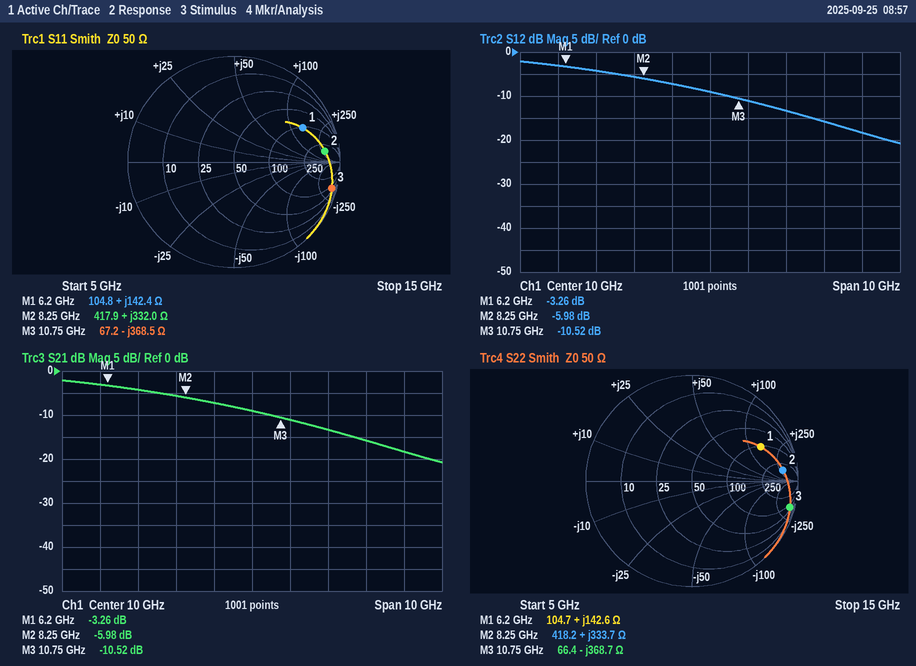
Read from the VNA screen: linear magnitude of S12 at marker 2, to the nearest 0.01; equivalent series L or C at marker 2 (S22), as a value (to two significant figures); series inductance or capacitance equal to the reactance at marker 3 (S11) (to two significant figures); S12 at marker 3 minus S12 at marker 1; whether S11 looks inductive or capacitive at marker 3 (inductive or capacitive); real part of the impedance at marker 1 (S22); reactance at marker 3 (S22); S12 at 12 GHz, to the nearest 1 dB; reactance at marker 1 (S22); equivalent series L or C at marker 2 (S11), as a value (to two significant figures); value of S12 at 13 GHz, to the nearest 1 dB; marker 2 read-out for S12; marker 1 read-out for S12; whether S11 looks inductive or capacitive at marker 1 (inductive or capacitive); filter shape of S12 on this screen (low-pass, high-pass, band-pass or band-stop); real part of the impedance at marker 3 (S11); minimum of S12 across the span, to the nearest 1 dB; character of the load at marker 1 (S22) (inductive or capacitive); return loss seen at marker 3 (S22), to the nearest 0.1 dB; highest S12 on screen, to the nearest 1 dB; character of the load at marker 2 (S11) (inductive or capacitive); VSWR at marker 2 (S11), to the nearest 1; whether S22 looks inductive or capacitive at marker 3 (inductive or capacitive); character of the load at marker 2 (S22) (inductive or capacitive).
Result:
0.50
6.4 nH
40 fF
-7.26 dB
capacitive
104.7 Ω
-368.7 Ω
-13 dB
+142.6 Ω
6.4 nH
-16 dB
-5.98 dB
-3.26 dB
inductive
low-pass
67.2 Ω
-21 dB
inductive
0.4 dB
-2 dB
inductive
14
capacitive
inductive
